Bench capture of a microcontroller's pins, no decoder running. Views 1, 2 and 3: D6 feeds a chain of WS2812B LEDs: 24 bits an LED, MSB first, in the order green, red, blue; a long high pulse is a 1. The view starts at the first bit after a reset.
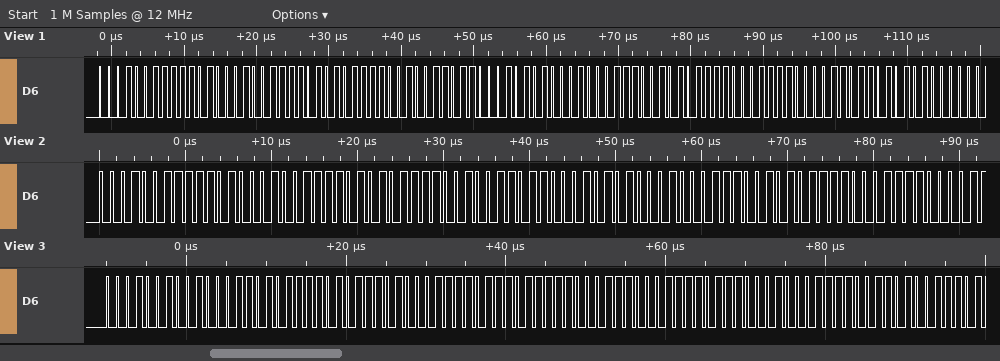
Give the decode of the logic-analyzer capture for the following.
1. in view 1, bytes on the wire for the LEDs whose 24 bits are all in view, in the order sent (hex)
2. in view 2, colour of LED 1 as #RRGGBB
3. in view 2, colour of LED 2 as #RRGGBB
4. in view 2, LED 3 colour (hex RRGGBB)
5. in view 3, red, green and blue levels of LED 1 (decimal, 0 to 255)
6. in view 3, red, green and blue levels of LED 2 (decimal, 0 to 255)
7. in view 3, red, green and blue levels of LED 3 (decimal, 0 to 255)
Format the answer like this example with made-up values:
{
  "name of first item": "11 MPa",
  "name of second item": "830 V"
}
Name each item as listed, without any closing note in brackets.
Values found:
{
  "in view 1, bytes on the wire for the LEDs whose 24 bits are all in view, in the order sent": "13 E8 9E AF 26 C5 44 72 BC 78 6D 50",
  "in view 2, colour of LED 1 as #RRGGBB": "#E8139E",
  "in view 2, colour of LED 2 as #RRGGBB": "#26AFC5",
  "in view 2, LED 3 colour": "#7244BC",
  "in view 3, red, green and blue levels of LED 1": "70, 18, 189",
  "in view 3, red, green and blue levels of LED 2": "123, 116, 190",
  "in view 3, red, green and blue levels of LED 3": "247, 56, 17"
}
